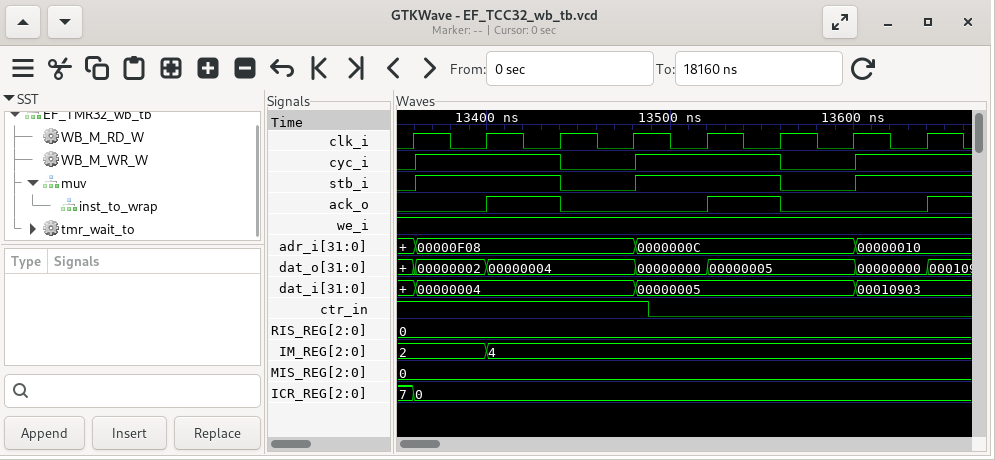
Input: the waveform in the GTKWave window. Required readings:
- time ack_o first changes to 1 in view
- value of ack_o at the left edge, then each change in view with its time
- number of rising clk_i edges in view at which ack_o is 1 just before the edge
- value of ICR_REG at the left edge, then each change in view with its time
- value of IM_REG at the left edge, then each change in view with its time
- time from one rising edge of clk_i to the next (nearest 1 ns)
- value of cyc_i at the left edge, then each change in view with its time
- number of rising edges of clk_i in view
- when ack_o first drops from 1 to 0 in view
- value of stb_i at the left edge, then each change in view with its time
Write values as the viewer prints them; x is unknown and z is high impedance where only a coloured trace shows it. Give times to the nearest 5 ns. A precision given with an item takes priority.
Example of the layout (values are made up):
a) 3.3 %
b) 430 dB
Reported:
a) 13400 ns
b) 0, 1 at 13400 ns, 0 at 13440 ns, 1 at 13520 ns, 0 at 13560 ns, 1 at 13640 ns
c) 2
d) 7, 0 at 13360 ns
e) 2, 4 at 13400 ns
f) 40 ns
g) 0, 1 at 13360 ns, 0 at 13440 ns, 1 at 13480 ns, 0 at 13560 ns, 1 at 13600 ns
h) 8
i) 13440 ns
j) 0, 1 at 13360 ns, 0 at 13440 ns, 1 at 13480 ns, 0 at 13560 ns, 1 at 13600 ns
